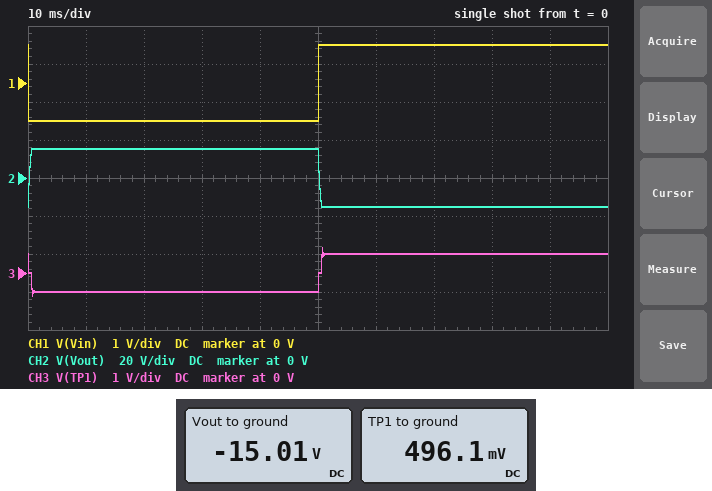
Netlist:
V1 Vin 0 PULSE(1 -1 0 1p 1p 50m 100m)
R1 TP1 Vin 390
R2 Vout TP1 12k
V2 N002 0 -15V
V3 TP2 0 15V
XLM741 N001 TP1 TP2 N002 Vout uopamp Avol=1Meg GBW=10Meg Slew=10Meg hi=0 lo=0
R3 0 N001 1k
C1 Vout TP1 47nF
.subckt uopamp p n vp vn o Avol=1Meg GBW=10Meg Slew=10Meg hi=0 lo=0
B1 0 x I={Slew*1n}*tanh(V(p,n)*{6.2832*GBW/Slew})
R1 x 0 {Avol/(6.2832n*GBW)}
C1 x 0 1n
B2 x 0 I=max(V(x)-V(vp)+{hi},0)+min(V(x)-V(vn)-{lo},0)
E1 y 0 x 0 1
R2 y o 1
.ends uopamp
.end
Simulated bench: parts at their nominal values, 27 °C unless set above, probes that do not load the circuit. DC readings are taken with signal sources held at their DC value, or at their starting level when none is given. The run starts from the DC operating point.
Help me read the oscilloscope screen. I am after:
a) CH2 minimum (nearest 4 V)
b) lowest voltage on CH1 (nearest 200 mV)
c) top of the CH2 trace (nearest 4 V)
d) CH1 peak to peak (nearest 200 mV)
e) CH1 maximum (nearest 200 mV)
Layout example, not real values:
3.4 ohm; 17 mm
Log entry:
-16 V; -1.0 V; 16 V; 2.0 V; 1.0 V
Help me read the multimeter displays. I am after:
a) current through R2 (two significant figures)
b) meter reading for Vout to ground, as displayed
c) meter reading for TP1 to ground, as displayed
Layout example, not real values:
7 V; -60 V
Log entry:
1.3 mA; -15.01 V; 496.1 mV
